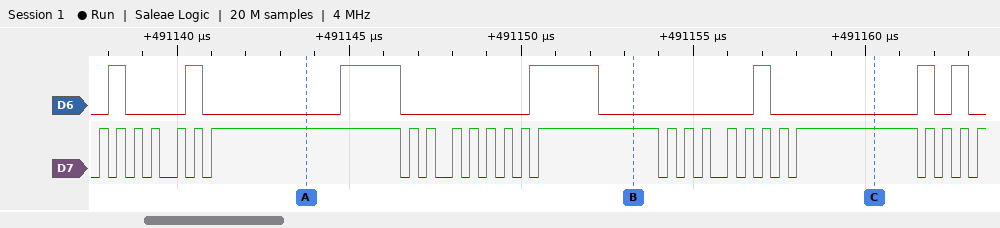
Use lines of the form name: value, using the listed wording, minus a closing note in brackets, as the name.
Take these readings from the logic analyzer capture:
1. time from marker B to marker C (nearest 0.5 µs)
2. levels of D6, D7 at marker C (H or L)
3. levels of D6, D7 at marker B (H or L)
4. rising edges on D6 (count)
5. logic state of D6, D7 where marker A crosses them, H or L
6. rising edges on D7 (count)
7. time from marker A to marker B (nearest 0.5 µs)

time from marker B to marker C: 7 µs
levels of D6, D7 at marker C: D6=L, D7=H
levels of D6, D7 at marker B: D6=L, D7=H
rising edges on D6: 7
logic state of D6, D7 where marker A crosses them, H or L: D6=L, D7=H
rising edges on D7: 27
time from marker A to marker B: 9.5 µs
